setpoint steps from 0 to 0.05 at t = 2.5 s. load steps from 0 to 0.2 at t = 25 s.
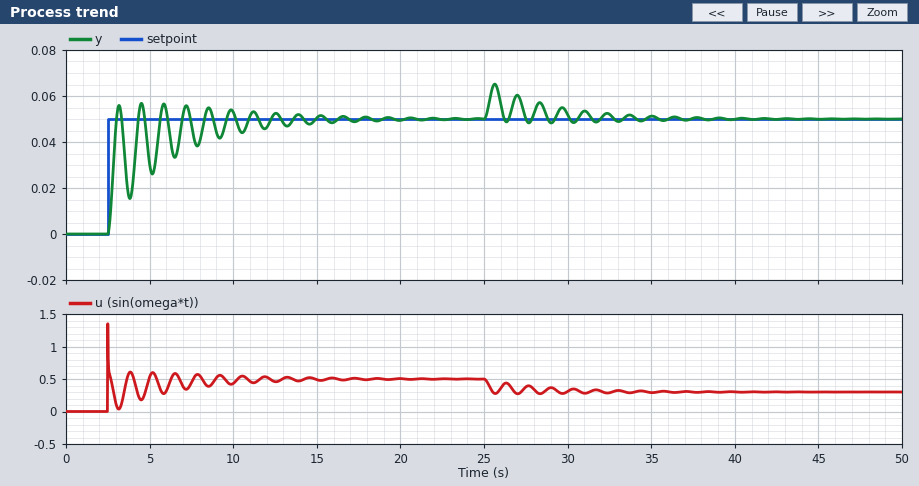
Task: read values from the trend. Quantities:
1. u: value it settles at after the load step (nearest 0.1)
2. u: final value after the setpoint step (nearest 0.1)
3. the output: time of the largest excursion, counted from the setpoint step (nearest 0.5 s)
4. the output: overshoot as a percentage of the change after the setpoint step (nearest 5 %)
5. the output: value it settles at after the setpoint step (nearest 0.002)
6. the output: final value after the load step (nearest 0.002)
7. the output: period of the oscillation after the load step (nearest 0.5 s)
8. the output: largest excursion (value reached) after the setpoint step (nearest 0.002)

0.3
0.5
2.0 s
15 %
0.050
0.050
1.5 s
0.056
